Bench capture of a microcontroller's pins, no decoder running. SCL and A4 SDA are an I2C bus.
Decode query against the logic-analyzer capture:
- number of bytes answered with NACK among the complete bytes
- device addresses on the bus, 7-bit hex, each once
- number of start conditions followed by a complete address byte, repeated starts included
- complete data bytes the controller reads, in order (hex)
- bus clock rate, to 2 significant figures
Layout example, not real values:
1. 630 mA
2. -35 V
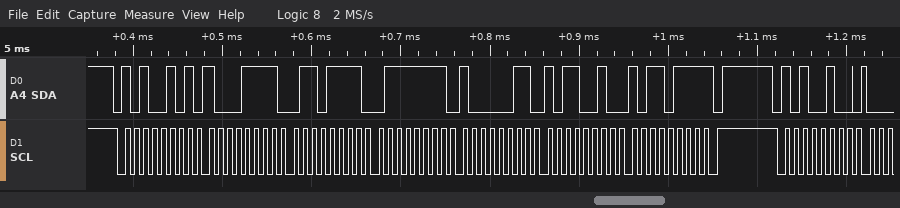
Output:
1. 1
2. 0x52
3. 2
4. 8F 6F 7F 83 B2 B7
5. 100 kHz
